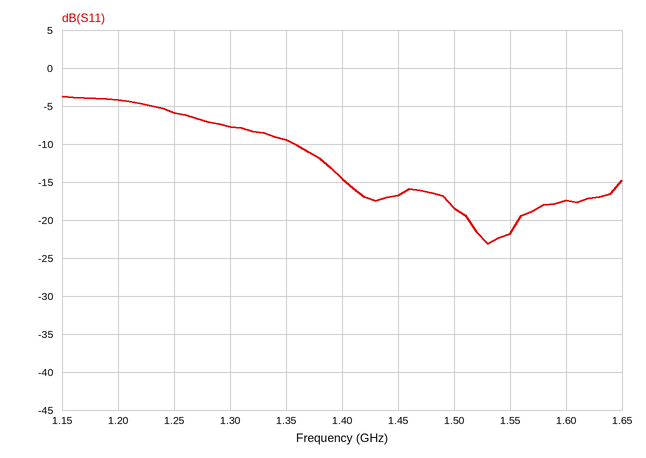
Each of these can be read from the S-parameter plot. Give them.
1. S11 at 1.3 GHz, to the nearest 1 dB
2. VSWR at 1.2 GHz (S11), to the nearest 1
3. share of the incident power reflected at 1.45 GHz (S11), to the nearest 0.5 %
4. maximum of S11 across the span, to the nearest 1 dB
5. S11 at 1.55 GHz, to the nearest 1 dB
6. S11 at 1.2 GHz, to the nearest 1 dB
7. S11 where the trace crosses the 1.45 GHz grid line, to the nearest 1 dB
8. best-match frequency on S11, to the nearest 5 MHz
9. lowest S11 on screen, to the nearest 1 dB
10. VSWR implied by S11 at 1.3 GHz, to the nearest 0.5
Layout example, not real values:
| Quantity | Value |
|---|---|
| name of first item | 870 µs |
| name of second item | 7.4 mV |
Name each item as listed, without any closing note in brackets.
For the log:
| Quantity | Value |
|---|---|
| S11 at 1.3 GHz, to the nearest 1 dB | -8 dB |
| VSWR at 1.2 GHz (S11), to the nearest 1 | 4 |
| share of the incident power reflected at 1.45 GHz (S11), to the nearest 0.5 % | 2.0 % |
| maximum of S11 across the span, to the nearest 1 dB | -4 dB |
| S11 at 1.55 GHz, to the nearest 1 dB | -22 dB |
| S11 at 1.2 GHz, to the nearest 1 dB | -4 dB |
| S11 where the trace crosses the 1.45 GHz grid line, to the nearest 1 dB | -17 dB |
| best-match frequency on S11, to the nearest 5 MHz | 1.530 GHz |
| lowest S11 on screen, to the nearest 1 dB | -23 dB |
| VSWR implied by S11 at 1.3 GHz, to the nearest 0.5 | 2.5 |
